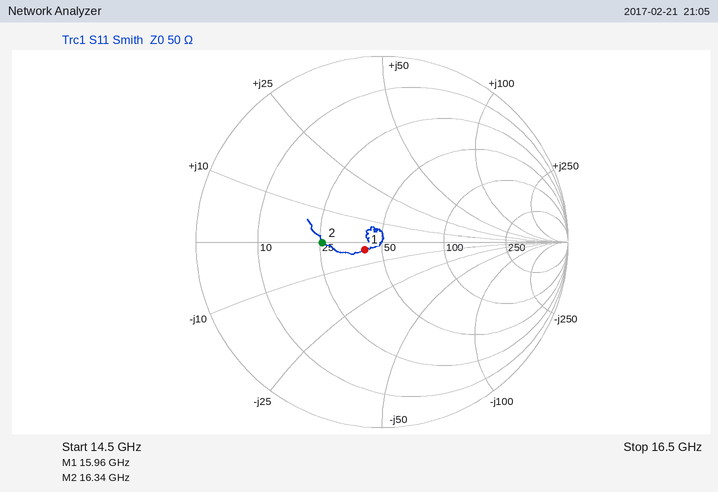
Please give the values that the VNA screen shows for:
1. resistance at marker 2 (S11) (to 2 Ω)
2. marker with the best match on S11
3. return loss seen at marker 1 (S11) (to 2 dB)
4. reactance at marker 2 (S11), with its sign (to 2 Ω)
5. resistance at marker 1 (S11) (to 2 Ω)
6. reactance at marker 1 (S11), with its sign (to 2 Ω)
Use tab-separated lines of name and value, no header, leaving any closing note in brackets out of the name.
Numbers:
resistance at marker 2 (S11)	26 Ω
marker with the best match on S11	marker 1
return loss seen at marker 1 (S11)	20 dB
reactance at marker 2 (S11), with its sign	0 Ω
resistance at marker 1 (S11)	42 Ω
reactance at marker 1 (S11), with its sign	-4 Ω
